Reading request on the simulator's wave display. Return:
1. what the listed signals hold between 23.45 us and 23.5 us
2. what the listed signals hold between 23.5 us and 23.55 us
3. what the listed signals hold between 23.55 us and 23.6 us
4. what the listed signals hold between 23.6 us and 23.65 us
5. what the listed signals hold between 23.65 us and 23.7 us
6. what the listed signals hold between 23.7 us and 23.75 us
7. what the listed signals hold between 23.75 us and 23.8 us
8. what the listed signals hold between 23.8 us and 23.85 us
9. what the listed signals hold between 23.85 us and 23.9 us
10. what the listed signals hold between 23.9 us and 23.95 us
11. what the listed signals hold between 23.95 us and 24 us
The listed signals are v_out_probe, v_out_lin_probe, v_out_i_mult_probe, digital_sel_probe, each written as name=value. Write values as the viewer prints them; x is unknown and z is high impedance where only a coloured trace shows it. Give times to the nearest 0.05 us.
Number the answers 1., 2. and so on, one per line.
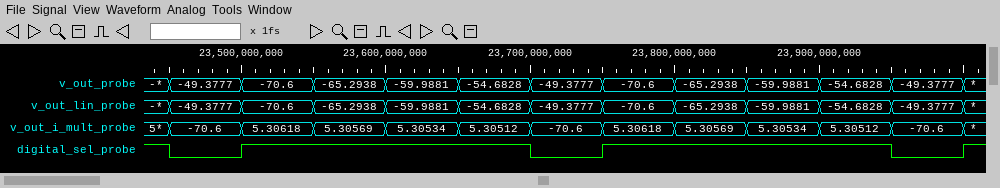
1. v_out_probe=-49.3777, v_out_lin_probe=-49.3777, v_out_i_mult_probe=-70.6, digital_sel_probe=0
2. v_out_probe=-70.6, v_out_lin_probe=-70.6, v_out_i_mult_probe=5.30618, digital_sel_probe=1
3. v_out_probe=-65.2938, v_out_lin_probe=-65.2938, v_out_i_mult_probe=5.30569, digital_sel_probe=1
4. v_out_probe=-59.9881, v_out_lin_probe=-59.9881, v_out_i_mult_probe=5.30534, digital_sel_probe=1
5. v_out_probe=-54.6828, v_out_lin_probe=-54.6828, v_out_i_mult_probe=5.30512, digital_sel_probe=1
6. v_out_probe=-49.3777, v_out_lin_probe=-49.3777, v_out_i_mult_probe=-70.6, digital_sel_probe=0
7. v_out_probe=-70.6, v_out_lin_probe=-70.6, v_out_i_mult_probe=5.30618, digital_sel_probe=1
8. v_out_probe=-65.2938, v_out_lin_probe=-65.2938, v_out_i_mult_probe=5.30569, digital_sel_probe=1
9. v_out_probe=-59.9881, v_out_lin_probe=-59.9881, v_out_i_mult_probe=5.30534, digital_sel_probe=1
10. v_out_probe=-54.6828, v_out_lin_probe=-54.6828, v_out_i_mult_probe=5.30512, digital_sel_probe=1
11. v_out_probe=-49.3777, v_out_lin_probe=-49.3777, v_out_i_mult_probe=-70.6, digital_sel_probe=0
